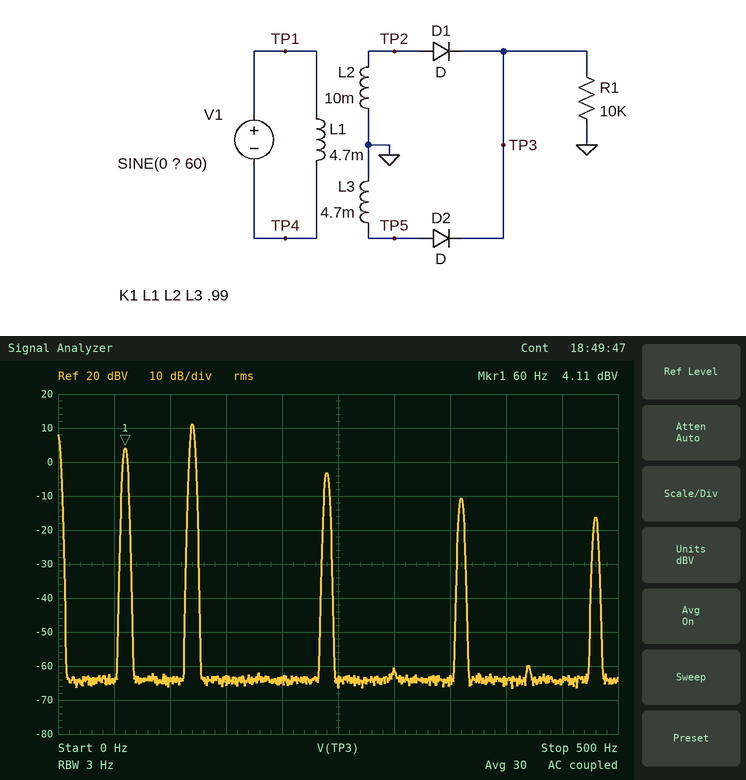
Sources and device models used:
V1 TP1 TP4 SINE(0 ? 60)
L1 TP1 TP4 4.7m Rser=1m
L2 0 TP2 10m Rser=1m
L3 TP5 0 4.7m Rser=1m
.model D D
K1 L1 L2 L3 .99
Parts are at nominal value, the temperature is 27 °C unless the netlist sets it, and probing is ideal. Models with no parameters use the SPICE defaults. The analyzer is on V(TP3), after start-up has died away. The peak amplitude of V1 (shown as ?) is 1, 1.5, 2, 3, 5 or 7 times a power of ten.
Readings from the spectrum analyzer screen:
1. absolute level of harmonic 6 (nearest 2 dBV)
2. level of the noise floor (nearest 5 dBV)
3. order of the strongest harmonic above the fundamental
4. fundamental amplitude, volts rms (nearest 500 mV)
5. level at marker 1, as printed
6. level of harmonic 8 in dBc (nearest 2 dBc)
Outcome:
-10 dBV
-65 dBV
2
1.5 V
4.11 dBV
-20 dBc
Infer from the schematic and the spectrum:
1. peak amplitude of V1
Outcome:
10 V
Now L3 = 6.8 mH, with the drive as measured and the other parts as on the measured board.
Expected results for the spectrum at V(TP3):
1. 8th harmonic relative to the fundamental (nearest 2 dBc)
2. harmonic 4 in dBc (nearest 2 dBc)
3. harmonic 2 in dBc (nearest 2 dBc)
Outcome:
-14 dBc
-2 dBc
12 dBc
